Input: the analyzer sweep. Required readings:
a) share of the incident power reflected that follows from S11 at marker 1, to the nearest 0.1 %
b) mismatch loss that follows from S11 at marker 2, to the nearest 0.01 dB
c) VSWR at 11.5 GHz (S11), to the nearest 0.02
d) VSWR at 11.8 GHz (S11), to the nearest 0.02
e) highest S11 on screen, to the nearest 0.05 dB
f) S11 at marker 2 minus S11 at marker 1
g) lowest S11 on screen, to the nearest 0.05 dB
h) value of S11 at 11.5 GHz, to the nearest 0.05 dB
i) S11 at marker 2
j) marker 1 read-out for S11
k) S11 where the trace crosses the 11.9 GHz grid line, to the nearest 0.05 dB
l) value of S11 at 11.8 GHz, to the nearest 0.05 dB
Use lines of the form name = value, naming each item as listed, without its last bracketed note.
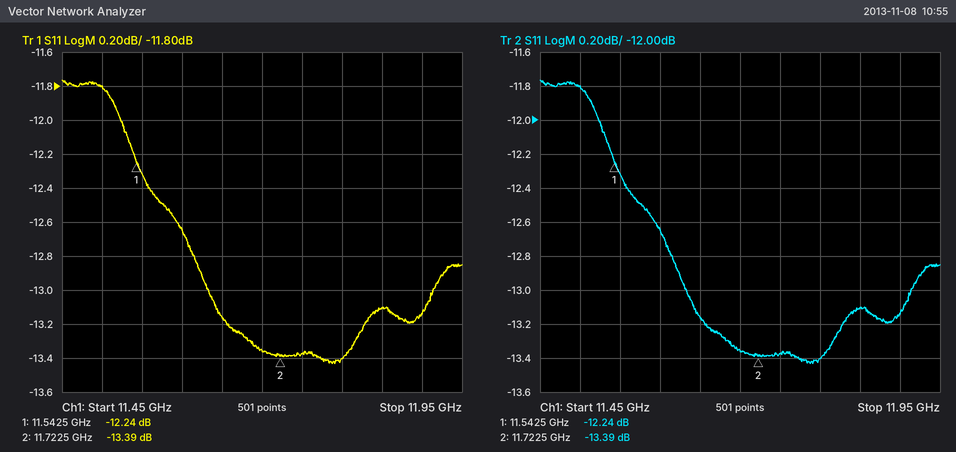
share of the incident power reflected that follows from S11 at marker 1, to the nearest 0.1 % = 6.0 %
mismatch loss that follows from S11 at marker 2, to the nearest 0.01 dB = 0.20 dB
VSWR at 11.5 GHz (S11), to the nearest 0.02 = 1.70
VSWR at 11.8 GHz (S11), to the nearest 0.02 = 1.54
highest S11 on screen, to the nearest 0.05 dB = -11.75 dB
S11 at marker 2 minus S11 at marker 1 = -1.15 dB
lowest S11 on screen, to the nearest 0.05 dB = -13.45 dB
value of S11 at 11.5 GHz, to the nearest 0.05 dB = -11.80 dB
S11 at marker 2 = -13.39 dB
marker 1 read-out for S11 = -12.24 dB
S11 where the trace crosses the 11.9 GHz grid line, to the nearest 0.05 dB = -13.15 dB
value of S11 at 11.8 GHz, to the nearest 0.05 dB = -13.40 dB
